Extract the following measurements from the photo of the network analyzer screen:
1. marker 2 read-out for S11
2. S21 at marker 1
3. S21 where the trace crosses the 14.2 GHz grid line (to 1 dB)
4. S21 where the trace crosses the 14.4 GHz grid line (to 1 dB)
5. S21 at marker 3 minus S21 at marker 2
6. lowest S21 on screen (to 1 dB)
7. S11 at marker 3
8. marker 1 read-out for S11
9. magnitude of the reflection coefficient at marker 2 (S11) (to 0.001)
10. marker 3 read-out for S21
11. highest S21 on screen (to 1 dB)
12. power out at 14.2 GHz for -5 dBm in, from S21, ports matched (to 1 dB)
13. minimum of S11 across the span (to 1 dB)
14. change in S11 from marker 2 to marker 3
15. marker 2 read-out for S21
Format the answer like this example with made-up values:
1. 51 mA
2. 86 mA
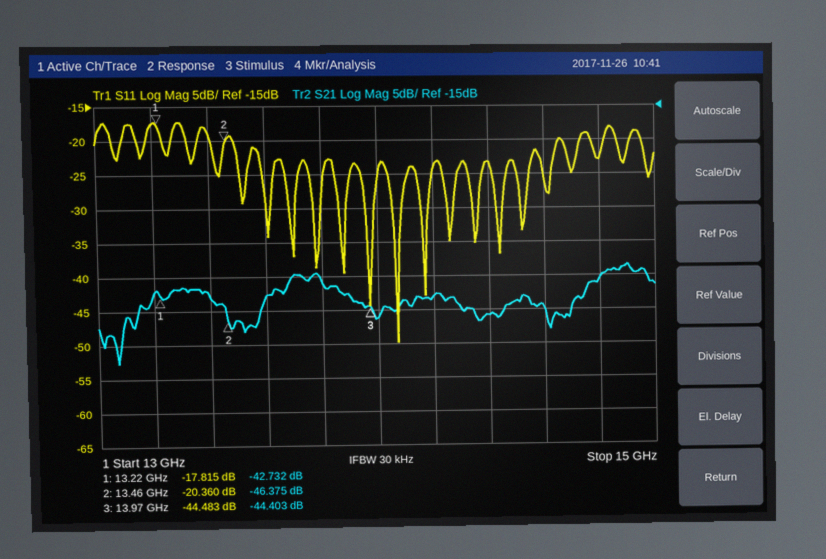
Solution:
1. -20.360 dB
2. -42.732 dB
3. -43 dB
4. -46 dB
5. 1.972 dB
6. -53 dB
7. -44.483 dB
8. -17.815 dB
9. 0.096
10. -44.403 dB
11. -38 dB
12. -48 dBm
13. -50 dB
14. -24.123 dB
15. -46.375 dB
